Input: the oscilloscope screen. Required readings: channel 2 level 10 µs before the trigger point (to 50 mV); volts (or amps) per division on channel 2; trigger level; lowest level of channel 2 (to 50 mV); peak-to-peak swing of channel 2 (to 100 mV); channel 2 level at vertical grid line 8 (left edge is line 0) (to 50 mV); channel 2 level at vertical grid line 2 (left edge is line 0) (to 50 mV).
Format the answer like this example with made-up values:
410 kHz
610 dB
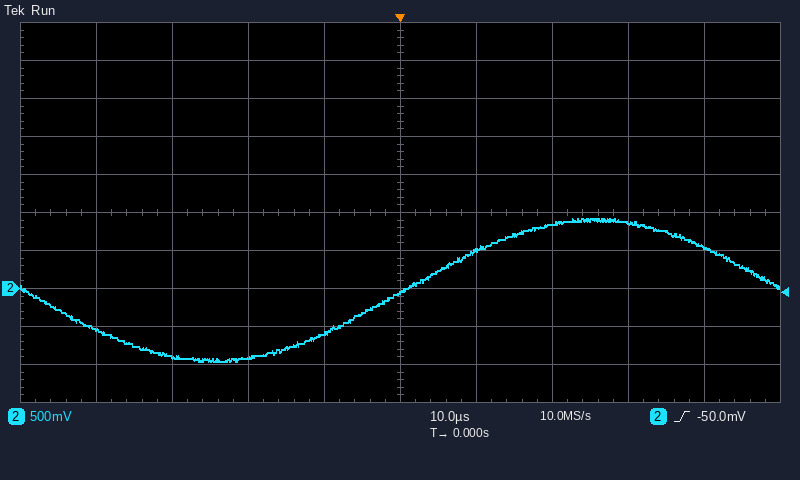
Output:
-600 mV
500 mV
-50.0 mV
-950 mV
1.90 V
850 mV
-900 mV
